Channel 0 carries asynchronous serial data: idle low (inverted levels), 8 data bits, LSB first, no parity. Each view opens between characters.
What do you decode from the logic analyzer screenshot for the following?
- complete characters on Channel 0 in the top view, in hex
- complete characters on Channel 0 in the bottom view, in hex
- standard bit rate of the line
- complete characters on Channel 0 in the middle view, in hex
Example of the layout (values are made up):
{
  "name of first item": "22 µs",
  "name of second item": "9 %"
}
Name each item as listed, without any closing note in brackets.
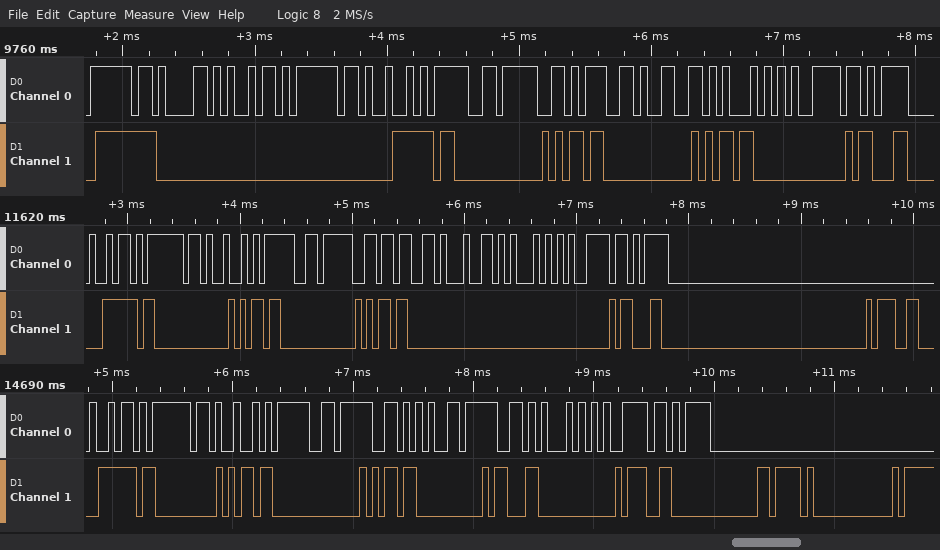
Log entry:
{
  "complete characters on Channel 0 in the top view, in hex": "20, 4F, 4B, 20, 5B, 30, 30, 31, 33, 5D, 0D, 0A",
  "complete characters on Channel 0 in the bottom view, in hex": "4B, 20, 5B, 30, 30, 35, 30, 5D, 0D, 0A",
  "standard bit rate of the line": "19200 baud",
  "complete characters on Channel 0 in the middle view, in hex": "4B, 20, 5B, 30, 30, 32, 37, 5D, 0D, 0A"
}
